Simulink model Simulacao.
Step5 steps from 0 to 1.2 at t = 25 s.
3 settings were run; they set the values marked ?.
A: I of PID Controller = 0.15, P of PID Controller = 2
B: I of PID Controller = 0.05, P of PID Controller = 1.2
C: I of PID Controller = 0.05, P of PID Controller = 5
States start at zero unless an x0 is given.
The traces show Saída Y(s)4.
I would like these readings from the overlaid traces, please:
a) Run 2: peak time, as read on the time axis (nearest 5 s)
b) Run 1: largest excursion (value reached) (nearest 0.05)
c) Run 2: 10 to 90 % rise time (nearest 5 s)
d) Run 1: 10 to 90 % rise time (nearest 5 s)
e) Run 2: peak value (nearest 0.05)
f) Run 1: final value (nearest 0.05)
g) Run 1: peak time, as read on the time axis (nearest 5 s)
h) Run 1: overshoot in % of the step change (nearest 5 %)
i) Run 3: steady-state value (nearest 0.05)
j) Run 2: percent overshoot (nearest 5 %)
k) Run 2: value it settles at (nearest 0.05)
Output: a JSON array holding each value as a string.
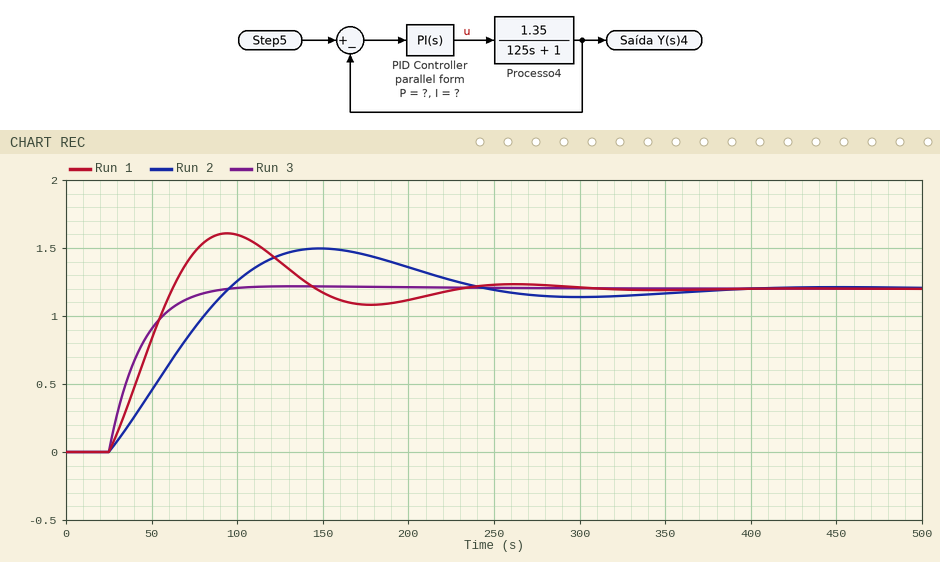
["150 s", "1.60", "55 s", "30 s", "1.50", "1.20", "95 s", "35 %", "1.20", "25 %", "1.20"]
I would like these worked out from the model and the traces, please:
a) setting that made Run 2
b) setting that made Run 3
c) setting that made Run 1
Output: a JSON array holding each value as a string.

["B", "C", "A"]
